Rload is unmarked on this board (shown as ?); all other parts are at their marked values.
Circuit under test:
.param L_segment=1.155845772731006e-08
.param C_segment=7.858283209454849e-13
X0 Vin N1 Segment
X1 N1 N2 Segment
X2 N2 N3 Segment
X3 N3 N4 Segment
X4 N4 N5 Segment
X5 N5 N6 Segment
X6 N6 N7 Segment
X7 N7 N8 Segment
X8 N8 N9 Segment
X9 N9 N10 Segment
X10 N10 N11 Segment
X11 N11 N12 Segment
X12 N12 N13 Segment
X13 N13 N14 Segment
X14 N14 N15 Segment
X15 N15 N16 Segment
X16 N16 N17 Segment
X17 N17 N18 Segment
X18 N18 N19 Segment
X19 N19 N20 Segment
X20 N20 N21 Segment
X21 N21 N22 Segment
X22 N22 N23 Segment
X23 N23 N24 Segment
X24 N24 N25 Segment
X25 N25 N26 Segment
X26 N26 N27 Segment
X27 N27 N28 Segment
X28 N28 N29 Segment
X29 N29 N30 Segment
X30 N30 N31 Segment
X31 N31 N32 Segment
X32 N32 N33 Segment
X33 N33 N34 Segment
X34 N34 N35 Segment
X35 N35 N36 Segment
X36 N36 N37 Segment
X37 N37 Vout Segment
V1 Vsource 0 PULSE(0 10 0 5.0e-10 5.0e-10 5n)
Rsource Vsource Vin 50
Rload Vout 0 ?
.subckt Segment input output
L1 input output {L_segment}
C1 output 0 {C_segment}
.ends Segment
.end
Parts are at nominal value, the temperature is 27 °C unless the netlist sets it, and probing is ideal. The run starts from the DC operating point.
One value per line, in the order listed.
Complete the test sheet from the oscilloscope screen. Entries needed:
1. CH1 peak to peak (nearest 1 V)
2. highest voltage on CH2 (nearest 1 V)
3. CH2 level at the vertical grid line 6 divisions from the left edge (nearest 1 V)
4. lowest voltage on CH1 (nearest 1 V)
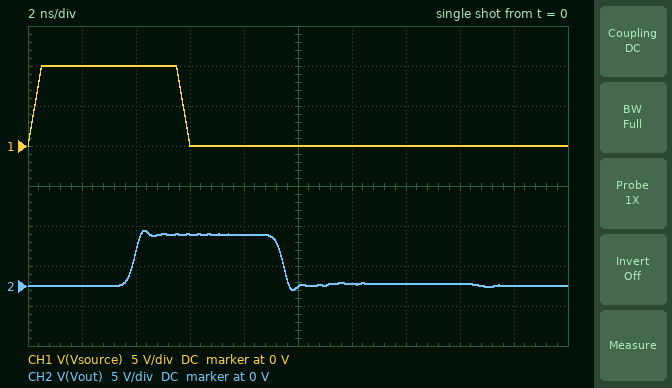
10 V
7 V
0 V
0 V
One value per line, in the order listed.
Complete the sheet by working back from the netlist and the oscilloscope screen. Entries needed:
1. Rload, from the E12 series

100 Ω
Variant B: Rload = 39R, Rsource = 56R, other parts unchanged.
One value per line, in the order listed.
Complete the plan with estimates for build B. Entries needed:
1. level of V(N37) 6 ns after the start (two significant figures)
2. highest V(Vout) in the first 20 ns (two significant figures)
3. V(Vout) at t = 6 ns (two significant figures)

3.2 V
3.6 V
3.3 V
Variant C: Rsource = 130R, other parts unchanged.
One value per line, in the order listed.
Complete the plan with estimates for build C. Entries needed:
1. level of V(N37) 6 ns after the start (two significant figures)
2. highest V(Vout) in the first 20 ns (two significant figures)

4.3 V
4.7 V
